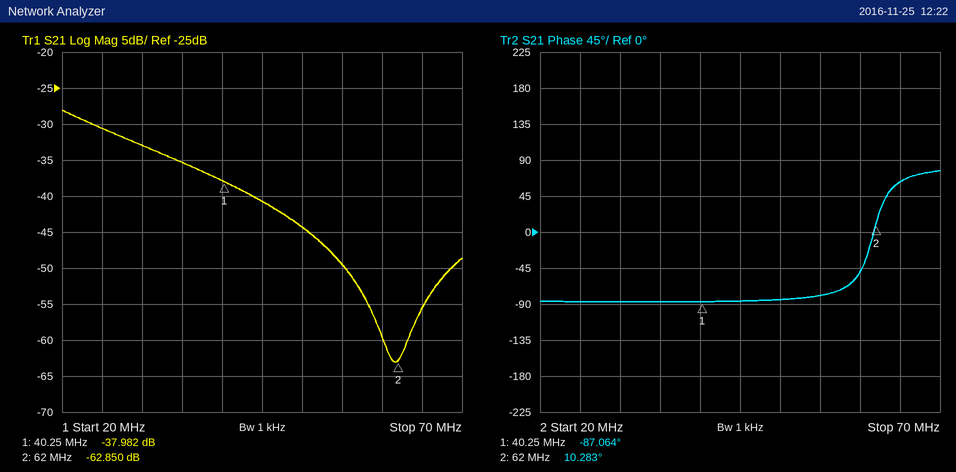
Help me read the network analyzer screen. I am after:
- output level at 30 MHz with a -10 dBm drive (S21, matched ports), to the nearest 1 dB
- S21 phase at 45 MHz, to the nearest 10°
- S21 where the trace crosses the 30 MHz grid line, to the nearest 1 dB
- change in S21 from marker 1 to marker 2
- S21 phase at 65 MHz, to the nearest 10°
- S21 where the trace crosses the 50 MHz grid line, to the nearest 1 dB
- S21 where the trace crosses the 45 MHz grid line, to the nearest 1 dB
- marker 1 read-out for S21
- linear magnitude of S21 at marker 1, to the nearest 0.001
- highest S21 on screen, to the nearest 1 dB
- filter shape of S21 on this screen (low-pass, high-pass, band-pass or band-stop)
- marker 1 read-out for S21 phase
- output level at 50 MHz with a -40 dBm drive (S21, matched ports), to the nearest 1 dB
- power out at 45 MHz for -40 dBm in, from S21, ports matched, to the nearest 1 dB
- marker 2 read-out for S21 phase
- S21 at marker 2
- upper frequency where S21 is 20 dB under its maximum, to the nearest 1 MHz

-43 dBm
-90°
-33 dB
-24.868 dB
60°
-44 dB
-41 dB
-37.982 dB
0.013
-28 dB
low-pass
-87.064°
-84 dBm
-81 dBm
10.283°
-62.850 dB
54 MHz
